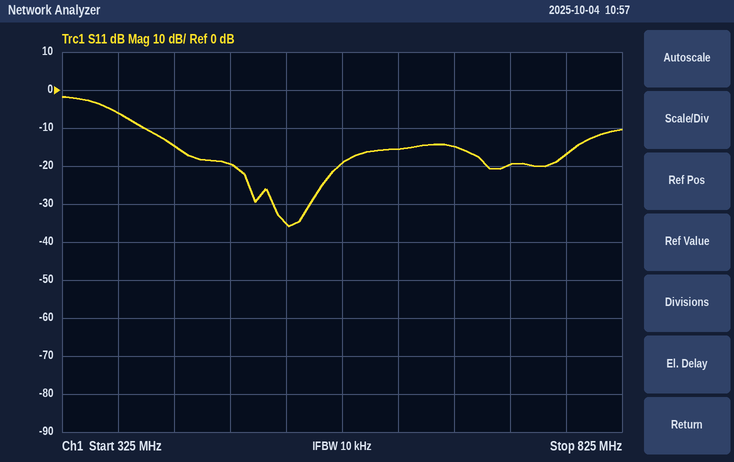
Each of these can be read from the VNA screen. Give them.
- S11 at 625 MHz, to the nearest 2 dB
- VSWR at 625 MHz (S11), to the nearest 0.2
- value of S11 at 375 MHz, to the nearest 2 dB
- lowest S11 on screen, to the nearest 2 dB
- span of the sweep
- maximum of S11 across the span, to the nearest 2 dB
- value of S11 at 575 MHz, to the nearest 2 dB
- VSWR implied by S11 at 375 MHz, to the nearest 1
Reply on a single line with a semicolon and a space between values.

-16 dB; 1.4; -6 dB; -36 dB; 500 MHz; -2 dB; -20 dB; 3
